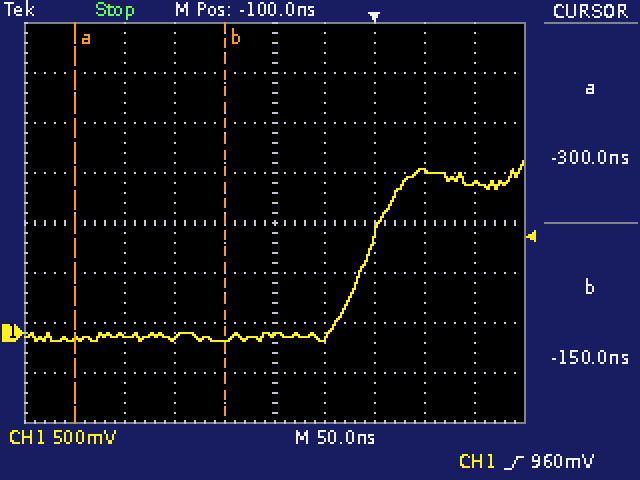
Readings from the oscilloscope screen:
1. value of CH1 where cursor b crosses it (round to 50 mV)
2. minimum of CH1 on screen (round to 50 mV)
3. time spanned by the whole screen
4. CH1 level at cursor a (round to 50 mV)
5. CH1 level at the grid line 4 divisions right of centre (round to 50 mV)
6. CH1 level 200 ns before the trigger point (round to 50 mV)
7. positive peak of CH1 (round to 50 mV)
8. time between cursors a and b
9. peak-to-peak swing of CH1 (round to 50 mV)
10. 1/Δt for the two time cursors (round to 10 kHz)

-50 mV
-100 mV
500 ns
-50 mV
1.50 V
-50 mV
1.70 V
150 ns
1.80 V
6.67 MHz
